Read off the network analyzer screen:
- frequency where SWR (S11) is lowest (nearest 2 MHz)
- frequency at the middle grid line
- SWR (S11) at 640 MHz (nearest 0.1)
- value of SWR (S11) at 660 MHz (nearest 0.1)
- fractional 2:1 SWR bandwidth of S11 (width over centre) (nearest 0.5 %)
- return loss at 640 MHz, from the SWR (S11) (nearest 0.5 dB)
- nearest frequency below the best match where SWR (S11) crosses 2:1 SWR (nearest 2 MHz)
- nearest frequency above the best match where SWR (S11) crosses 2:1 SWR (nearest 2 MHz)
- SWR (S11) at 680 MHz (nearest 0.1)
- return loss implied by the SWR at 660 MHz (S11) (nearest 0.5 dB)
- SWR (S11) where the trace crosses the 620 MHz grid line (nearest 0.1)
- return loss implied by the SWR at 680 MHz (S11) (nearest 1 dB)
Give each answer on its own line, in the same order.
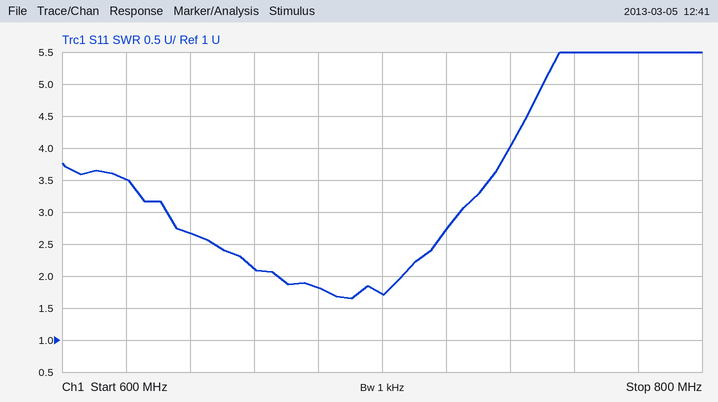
690 MHz
700 MHz
2.7
2.1
5.5 %
7.0 dB
668 MHz
706 MHz
1.8
9.0 dB
3.5
11 dB
